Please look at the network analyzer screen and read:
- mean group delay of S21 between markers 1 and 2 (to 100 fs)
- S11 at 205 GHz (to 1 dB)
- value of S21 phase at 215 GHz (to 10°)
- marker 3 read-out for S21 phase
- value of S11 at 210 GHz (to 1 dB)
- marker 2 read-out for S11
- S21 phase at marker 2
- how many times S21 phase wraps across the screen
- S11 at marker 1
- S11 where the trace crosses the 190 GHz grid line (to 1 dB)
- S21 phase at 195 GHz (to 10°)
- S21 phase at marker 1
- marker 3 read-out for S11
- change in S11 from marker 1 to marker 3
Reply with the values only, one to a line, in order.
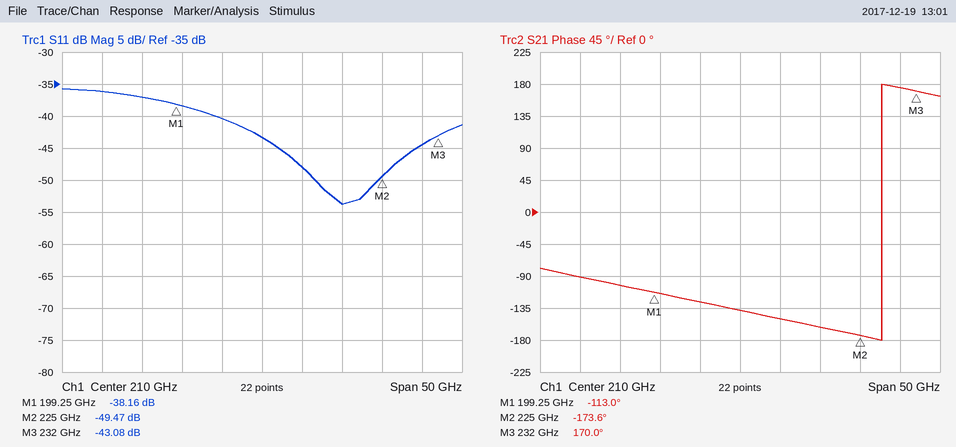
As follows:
6.5 ps
-40 dB
-150°
170.0°
-43 dB
-49.47 dB
-173.6°
1
-38.16 dB
-36 dB
-100°
-113.0°
-43.08 dB
-4.92 dB
